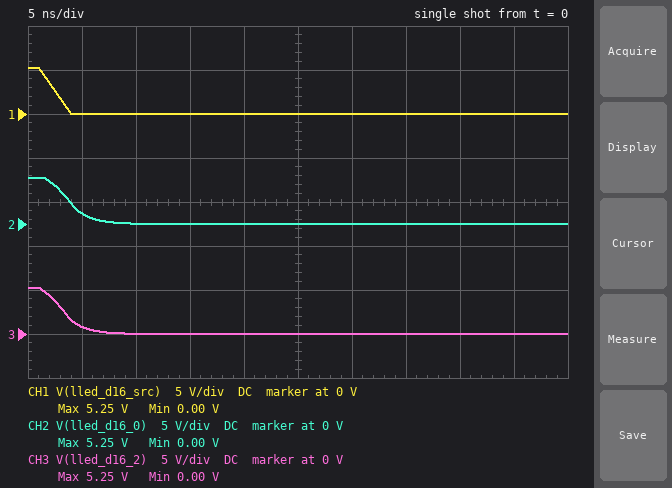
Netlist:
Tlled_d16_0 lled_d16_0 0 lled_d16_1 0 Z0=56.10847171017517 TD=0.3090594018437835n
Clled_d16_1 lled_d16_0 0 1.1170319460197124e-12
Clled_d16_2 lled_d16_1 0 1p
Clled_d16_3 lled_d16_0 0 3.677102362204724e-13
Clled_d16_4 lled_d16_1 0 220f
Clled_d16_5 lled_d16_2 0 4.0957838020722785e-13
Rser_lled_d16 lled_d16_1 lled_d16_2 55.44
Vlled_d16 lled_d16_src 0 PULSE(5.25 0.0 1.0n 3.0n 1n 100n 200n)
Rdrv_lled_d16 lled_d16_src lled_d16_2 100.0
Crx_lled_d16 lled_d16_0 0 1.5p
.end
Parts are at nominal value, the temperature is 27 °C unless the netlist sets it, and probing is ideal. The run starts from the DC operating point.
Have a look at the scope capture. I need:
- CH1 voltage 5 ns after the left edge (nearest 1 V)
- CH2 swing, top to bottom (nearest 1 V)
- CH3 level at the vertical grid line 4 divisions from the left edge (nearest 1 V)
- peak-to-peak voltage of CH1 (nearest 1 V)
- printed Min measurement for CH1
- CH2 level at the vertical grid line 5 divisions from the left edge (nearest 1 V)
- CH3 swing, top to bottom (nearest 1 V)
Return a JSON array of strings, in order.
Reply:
["0 V", "5 V", "0 V", "5 V", "0.00 V", "0 V", "5 V"]
